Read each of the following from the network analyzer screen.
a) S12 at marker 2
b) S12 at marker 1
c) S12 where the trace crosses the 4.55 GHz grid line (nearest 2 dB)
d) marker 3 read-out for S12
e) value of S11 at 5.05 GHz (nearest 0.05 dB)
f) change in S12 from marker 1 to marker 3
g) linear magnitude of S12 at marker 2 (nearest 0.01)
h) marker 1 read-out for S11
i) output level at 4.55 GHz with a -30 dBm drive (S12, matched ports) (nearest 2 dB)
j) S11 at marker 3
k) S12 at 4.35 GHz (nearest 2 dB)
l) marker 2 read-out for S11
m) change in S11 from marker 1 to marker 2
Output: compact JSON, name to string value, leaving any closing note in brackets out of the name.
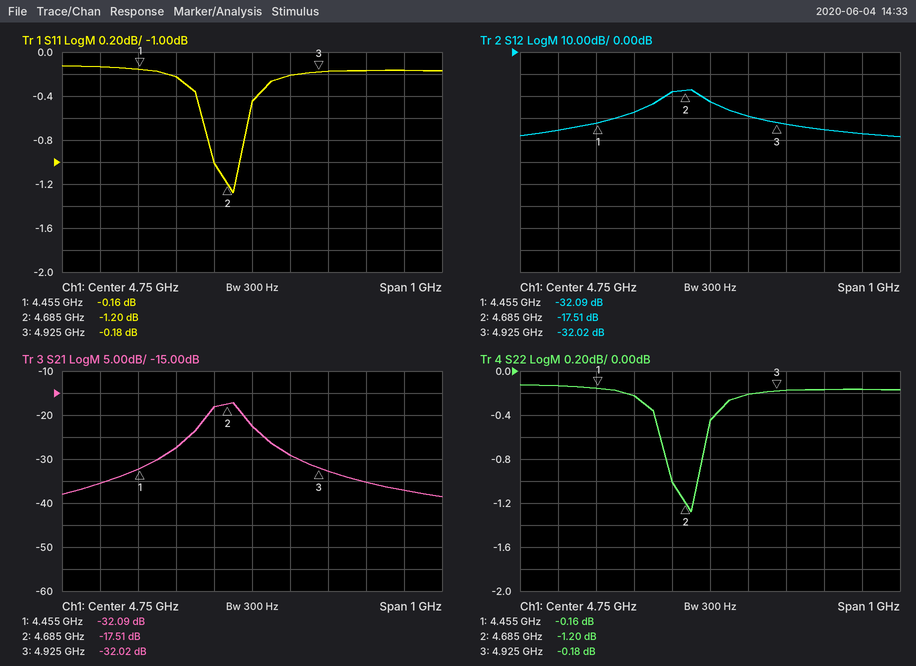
{"S12 at marker 2": "-17.51 dB", "S12 at marker 1": "-32.09 dB", "S12 where the trace crosses the 4.55 GHz grid line": "-28 dB", "marker 3 read-out for S12": "-32.02 dB", "value of S11 at 5.05 GHz": "-0.15 dB", "change in S12 from marker 1 to marker 3": "0.07 dB", "linear magnitude of S12 at marker 2": "0.13", "marker 1 read-out for S11": "-0.16 dB", "output level at 4.55 GHz with a -30 dBm drive (S12, matched ports)": "-58 dBm", "S11 at marker 3": "-0.18 dB", "S12 at 4.35 GHz": "-36 dB", "marker 2 read-out for S11": "-1.20 dB", "change in S11 from marker 1 to marker 2": "-1.04 dB"}
